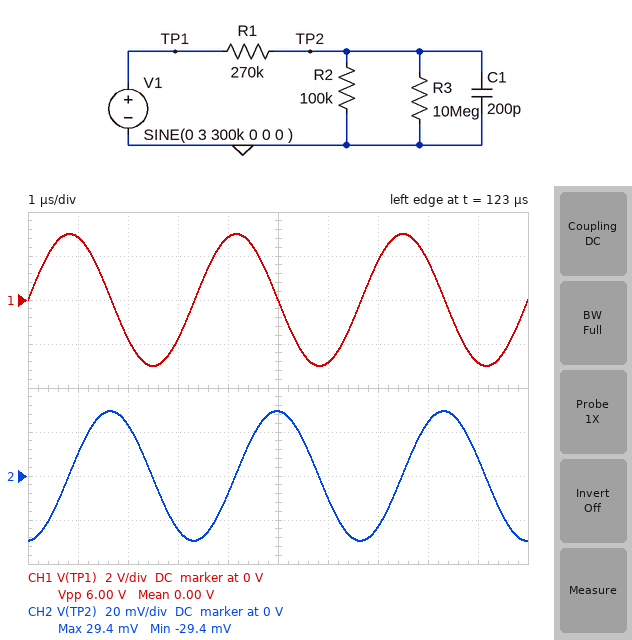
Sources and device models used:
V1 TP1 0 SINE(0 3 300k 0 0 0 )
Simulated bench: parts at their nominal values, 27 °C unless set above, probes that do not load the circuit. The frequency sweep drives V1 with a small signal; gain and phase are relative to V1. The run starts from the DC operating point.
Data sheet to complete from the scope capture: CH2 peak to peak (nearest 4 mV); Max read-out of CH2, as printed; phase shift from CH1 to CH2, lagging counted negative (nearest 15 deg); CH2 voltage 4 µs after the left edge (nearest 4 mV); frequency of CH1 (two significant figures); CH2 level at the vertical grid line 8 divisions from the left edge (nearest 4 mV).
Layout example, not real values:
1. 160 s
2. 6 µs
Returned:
1. 60 mV
2. 29.4 mV
3. -90 deg
4. -8 mV
5. 300 kHz
6. 24 mV
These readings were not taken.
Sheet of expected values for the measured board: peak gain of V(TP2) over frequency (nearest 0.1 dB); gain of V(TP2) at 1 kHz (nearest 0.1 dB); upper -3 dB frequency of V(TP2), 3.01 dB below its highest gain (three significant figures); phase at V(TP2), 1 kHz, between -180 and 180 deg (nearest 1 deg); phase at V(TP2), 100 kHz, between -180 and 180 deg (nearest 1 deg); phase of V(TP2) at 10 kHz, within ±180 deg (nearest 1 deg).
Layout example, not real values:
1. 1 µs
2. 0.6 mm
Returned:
1. -11.4 dB
2. -11.5 dB
3. 11.0 kHz
4. -5 deg
5. -84 deg
6. -42 deg
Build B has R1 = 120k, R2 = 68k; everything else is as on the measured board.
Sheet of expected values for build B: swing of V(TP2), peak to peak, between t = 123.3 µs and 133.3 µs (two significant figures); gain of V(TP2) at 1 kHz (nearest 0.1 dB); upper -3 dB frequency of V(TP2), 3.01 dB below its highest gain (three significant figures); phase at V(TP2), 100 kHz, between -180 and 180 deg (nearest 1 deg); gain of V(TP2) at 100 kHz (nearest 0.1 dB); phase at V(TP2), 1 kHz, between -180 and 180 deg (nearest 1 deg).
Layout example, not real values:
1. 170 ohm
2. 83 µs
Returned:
1. 130 mV
2. -8.9 dB
3. 18.4 kHz
4. -80 deg
5. -23.7 dB
6. -3 deg
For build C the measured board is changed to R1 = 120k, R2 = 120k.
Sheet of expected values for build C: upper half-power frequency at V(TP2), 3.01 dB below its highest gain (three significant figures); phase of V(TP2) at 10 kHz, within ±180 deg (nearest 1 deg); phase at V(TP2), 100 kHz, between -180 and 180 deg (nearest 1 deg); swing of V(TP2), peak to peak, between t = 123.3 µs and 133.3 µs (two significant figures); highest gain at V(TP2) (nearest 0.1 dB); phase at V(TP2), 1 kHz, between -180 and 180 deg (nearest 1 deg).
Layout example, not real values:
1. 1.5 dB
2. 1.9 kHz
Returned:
1. 13.3 kHz
2. -37 deg
3. -82 deg
4. 130 mV
5. -6.1 dB
6. -4 deg
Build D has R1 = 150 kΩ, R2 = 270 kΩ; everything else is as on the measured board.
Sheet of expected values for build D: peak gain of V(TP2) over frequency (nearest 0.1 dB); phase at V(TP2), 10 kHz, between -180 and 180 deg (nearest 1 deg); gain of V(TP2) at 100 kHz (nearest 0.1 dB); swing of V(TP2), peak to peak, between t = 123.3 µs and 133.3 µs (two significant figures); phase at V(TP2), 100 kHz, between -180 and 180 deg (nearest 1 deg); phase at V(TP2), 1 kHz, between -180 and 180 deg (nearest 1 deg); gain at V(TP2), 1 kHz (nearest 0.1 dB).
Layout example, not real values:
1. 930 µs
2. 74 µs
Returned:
1. -3.9 dB
2. -50 deg
3. -25.5 dB
4. 110 mV
5. -85 deg
6. -7 deg
7. -4.0 dB
